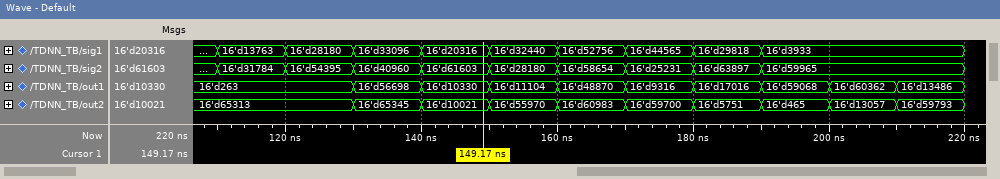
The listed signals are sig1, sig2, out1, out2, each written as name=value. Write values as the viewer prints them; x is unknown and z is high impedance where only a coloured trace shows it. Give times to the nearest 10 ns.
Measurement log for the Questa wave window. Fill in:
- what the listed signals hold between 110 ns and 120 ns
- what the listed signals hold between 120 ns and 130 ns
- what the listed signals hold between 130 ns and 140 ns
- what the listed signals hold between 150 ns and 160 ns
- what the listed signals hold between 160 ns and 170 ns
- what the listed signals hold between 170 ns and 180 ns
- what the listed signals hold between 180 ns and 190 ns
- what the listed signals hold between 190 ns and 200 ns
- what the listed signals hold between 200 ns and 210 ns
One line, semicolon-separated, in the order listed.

sig1=16'd13763, sig2=16'd31784, out1=16'd263, out2=16'd65313; sig1=16'd28180, sig2=16'd54395, out1=16'd263, out2=16'd65313; sig1=16'd33096, sig2=16'd40960, out1=16'd56698, out2=16'd65345; sig1=16'd32440, sig2=16'd28180, out1=16'd11104, out2=16'd55970; sig1=16'd52756, sig2=16'd58654, out1=16'd48870, out2=16'd60983; sig1=16'd44565, sig2=16'd25231, out1=16'd9316, out2=16'd59700; sig1=16'd29818, sig2=16'd63897, out1=16'd17016, out2=16'd5751; sig1=16'd3933, sig2=16'd59965, out1=16'd59068, out2=16'd465; sig1=16'd3933, sig2=16'd59965, out1=16'd60362, out2=16'd13057
